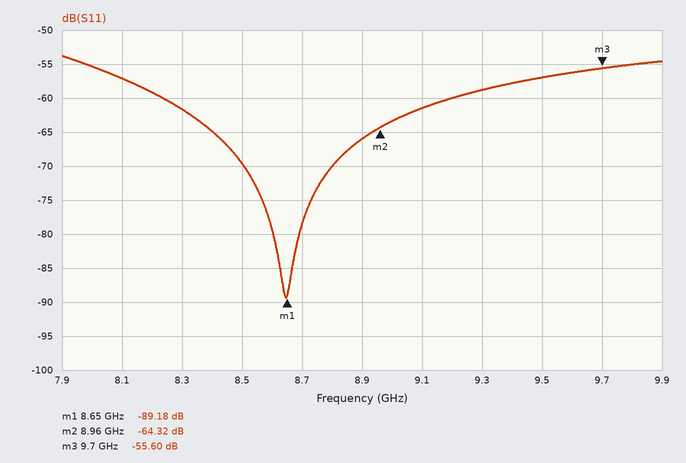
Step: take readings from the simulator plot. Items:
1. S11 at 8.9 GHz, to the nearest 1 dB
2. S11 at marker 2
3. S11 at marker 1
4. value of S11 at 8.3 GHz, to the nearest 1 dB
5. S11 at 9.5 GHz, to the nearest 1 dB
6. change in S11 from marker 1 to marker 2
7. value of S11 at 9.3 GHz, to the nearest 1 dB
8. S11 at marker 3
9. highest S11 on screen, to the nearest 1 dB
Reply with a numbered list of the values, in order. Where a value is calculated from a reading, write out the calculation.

1. -66 dB
2. -64.32 dB
3. -89.18 dB
4. -62 dB
5. -57 dB
6. -64.32 − (-89.18) = 24.86 dB
7. -59 dB
8. -55.60 dB
9. -54 dB
